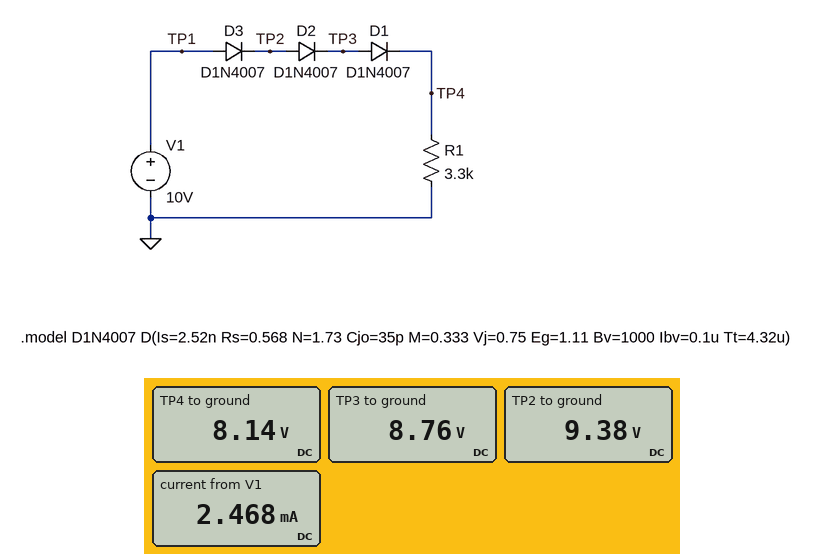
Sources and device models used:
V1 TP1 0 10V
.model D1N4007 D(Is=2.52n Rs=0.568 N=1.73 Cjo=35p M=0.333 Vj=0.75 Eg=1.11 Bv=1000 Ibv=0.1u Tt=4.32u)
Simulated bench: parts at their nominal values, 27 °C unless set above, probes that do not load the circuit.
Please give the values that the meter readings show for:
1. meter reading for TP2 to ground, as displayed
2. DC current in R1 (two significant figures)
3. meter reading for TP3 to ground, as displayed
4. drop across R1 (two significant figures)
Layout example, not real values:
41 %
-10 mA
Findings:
9.38 V
2.5 mA
8.76 V
8.1 V
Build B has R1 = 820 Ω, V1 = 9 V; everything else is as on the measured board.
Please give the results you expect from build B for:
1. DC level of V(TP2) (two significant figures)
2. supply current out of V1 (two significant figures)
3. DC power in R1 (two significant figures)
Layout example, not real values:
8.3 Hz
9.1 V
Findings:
8.3 V
8.5 mA
59 mW
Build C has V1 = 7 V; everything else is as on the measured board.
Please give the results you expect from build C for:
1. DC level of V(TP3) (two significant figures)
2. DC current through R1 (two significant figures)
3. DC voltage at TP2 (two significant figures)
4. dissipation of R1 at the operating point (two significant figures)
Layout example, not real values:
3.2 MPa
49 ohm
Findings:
5.8 V
1.6 mA
6.4 V
8.2 mW
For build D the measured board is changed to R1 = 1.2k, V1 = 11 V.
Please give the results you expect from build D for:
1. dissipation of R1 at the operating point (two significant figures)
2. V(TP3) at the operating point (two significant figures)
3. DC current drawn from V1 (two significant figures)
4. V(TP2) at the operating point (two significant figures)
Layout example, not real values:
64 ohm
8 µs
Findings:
67 mW
9.7 V
7.5 mA
10 V
